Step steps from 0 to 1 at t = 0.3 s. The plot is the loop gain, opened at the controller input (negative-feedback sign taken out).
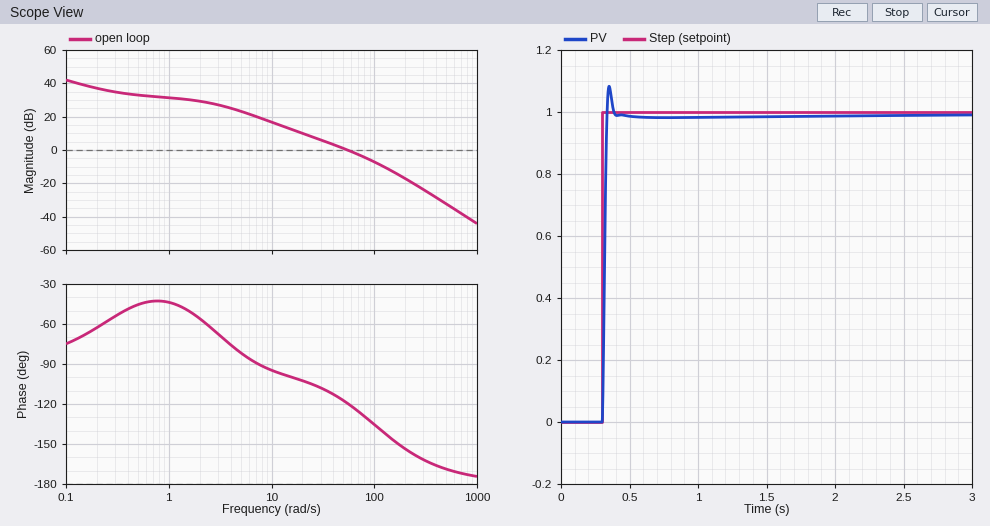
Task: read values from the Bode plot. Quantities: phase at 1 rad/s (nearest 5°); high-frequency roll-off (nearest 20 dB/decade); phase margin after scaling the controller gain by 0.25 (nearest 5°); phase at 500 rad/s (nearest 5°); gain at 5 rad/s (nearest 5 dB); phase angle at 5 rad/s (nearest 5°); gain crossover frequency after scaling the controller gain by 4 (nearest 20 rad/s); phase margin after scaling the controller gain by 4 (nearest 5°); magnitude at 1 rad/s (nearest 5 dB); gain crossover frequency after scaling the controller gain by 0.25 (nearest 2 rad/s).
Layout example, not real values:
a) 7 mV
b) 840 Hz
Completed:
a) -45°
b) -40 dB/decade
c) 80°
d) -170°
e) 25 dB
f) -80°
g) 140 rad/s
h) 35°
i) 30 dB
j) 16 rad/s
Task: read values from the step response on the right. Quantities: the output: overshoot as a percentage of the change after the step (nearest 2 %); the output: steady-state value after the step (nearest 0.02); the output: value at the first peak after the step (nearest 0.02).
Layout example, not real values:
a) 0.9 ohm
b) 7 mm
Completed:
a) 8 %
b) 1.00
c) 1.08
